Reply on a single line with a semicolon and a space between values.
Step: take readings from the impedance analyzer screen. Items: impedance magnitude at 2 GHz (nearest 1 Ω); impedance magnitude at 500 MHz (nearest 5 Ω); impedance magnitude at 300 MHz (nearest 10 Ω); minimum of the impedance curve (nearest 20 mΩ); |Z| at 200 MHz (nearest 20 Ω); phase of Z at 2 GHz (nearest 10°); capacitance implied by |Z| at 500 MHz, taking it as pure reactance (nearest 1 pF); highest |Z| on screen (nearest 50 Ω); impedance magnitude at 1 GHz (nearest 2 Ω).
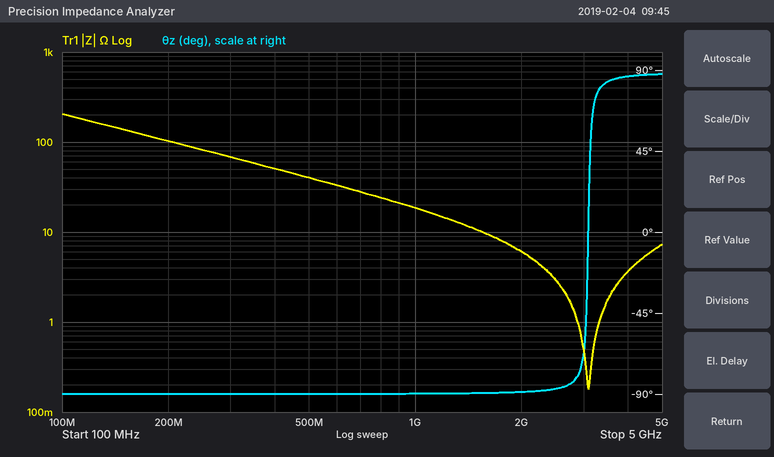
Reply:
6 Ω; 40 Ω; 70 Ω; 180 mΩ; 100 Ω; -90°; 8 pF; 200 Ω; 18 Ω
